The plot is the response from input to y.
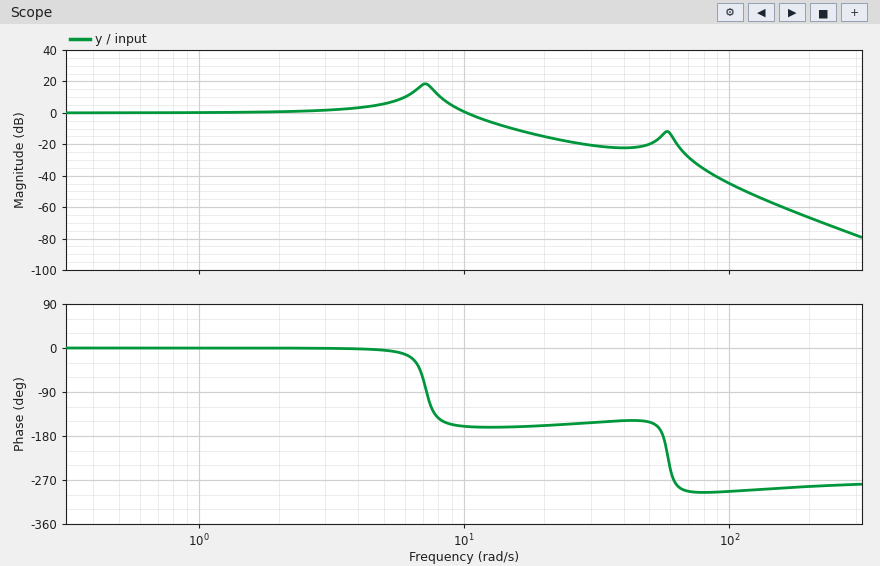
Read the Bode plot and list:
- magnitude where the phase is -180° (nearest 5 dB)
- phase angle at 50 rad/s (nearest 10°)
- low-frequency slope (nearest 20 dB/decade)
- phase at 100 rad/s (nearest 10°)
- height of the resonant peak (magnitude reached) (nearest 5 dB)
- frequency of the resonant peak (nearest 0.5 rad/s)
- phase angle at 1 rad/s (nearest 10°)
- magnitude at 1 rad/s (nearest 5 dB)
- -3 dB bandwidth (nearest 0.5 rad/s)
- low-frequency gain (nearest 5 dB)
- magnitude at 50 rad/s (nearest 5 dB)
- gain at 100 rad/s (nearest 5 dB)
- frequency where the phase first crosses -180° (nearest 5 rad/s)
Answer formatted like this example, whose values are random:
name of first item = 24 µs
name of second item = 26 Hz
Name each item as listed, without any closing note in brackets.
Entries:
magnitude where the phase is -180° = -15 dB
phase angle at 50 rad/s = -150°
low-frequency slope = 0 dB/decade
phase at 100 rad/s = -290°
height of the resonant peak (magnitude reached) = 20 dB
frequency of the resonant peak = 7.0 rad/s
phase angle at 1 rad/s = 0°
magnitude at 1 rad/s = 0 dB
-3 dB bandwidth = 11.5 rad/s
low-frequency gain = 0 dB
magnitude at 50 rad/s = -20 dB
gain at 100 rad/s = -45 dB
frequency where the phase first crosses -180° = 55 rad/s
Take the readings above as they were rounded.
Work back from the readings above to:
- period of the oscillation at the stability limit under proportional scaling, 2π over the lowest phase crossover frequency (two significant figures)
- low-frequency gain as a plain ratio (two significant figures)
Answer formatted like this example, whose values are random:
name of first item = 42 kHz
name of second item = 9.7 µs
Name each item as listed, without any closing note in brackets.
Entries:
period of the oscillation at the stability limit under proportional scaling, 2π over the lowest phase crossover frequency = 0.11 s
low-frequency gain as a plain ratio = 1.0
